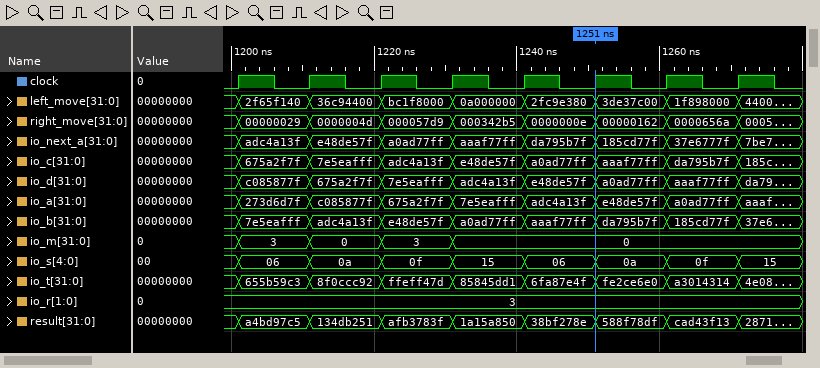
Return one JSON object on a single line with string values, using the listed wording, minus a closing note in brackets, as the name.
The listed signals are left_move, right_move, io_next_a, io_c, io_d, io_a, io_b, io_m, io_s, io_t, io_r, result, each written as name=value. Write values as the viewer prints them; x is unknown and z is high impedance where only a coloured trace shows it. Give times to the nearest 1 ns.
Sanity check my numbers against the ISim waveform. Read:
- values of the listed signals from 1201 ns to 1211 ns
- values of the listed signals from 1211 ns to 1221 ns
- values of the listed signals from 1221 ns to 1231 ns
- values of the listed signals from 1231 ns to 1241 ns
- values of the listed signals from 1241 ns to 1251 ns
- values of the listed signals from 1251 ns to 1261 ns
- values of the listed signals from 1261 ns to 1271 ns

{"values of the listed signals from 1201 ns to 1211 ns": "left_move=2f65f140, right_move=00000029, io_next_a=adc4a13f, io_c=675a2f7f, io_d=c085877f, io_a=273d6d7f, io_b=7e5eafff, io_m=3, io_s=06, io_t=655b59c3, io_r=3, result=a4bd97c5", "values of the listed signals from 1211 ns to 1221 ns": "left_move=36c94400, right_move=0000004d, io_next_a=e48de57f, io_c=7e5eafff, io_d=675a2f7f, io_a=c085877f, io_b=adc4a13f, io_m=0, io_s=0a, io_t=8f0ccc92, io_r=3, result=134db251", "values of the listed signals from 1221 ns to 1231 ns": "left_move=bc1f8000, right_move=000057d9, io_next_a=a0ad77ff, io_c=adc4a13f, io_d=7e5eafff, io_a=675a2f7f, io_b=e48de57f, io_m=3, io_s=0f, io_t=ffeff47d, io_r=3, result=afb3783f", "values of the listed signals from 1231 ns to 1241 ns": "left_move=0a000000, right_move=000342b5, io_next_a=aaaf77ff, io_c=e48de57f, io_d=adc4a13f, io_a=7e5eafff, io_b=a0ad77ff, io_m=0, io_s=15, io_t=85845dd1, io_r=3, result=1a15a850", "values of the listed signals from 1241 ns to 1251 ns": "left_move=2fc9e380, right_move=0000000e, io_next_a=da795b7f, io_c=a0ad77ff, io_d=e48de57f, io_a=adc4a13f, io_b=aaaf77ff, io_m=0, io_s=06, io_t=6fa87e4f, io_r=3, result=38bf278e", "values of the listed signals from 1251 ns to 1261 ns": "left_move=3de37c00, right_move=00000162, io_next_a=185cd77f, io_c=aaaf77ff, io_d=a0ad77ff, io_a=e48de57f, io_b=da795b7f, io_m=0, io_s=0a, io_t=fe2ce6e0, io_r=3, result=588f78df", "values of the listed signals from 1261 ns to 1271 ns": "left_move=1f898000, right_move=0000656a, io_next_a=37e6777f, io_c=da795b7f, io_d=aaaf77ff, io_a=a0ad77ff, io_b=185cd77f, io_m=0, io_s=0f, io_t=a3014314, io_r=3, result=cad43f13"}
